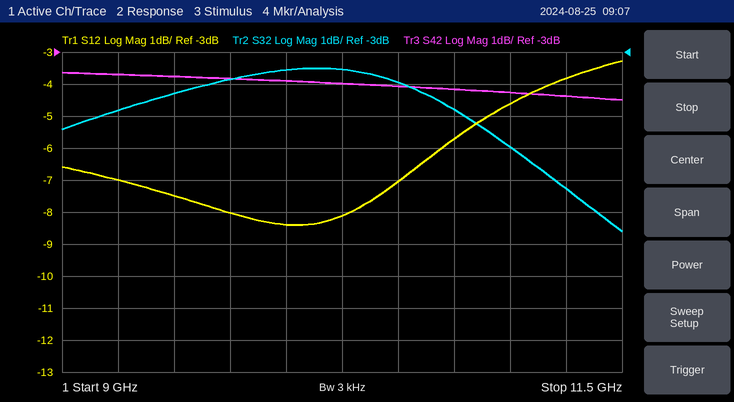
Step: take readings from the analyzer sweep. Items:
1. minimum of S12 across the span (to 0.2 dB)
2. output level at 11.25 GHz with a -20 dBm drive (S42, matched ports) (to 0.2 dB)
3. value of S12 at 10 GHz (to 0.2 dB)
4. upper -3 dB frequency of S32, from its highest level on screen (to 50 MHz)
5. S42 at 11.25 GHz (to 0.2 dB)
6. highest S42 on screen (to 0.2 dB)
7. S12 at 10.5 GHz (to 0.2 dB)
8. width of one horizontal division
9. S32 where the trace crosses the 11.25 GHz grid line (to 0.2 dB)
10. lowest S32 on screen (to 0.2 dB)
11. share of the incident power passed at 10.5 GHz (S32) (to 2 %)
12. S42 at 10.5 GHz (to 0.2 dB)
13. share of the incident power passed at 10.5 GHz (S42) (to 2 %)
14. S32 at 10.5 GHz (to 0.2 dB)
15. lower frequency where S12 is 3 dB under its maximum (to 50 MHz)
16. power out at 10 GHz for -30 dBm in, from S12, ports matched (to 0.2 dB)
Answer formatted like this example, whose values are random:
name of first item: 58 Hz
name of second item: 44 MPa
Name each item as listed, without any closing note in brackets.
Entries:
minimum of S12 across the span: -8.4 dB
output level at 11.25 GHz with a -20 dBm drive (S42, matched ports): -24.4 dBm
value of S12 at 10 GHz: -8.4 dB
upper -3 dB frequency of S32, from its highest level on screen: 11.10 GHz
S42 at 11.25 GHz: -4.4 dB
highest S42 on screen: -3.6 dB
S12 at 10.5 GHz: -7.0 dB
width of one horizontal division: 250 MHz
S32 where the trace crosses the 11.25 GHz grid line: -7.2 dB
lowest S32 on screen: -8.6 dB
share of the incident power passed at 10.5 GHz (S32): 40 %
S42 at 10.5 GHz: -4.0 dB
share of the incident power passed at 10.5 GHz (S42): 40 %
S32 at 10.5 GHz: -4.0 dB
lower frequency where S12 is 3 dB under its maximum: 10.65 GHz
power out at 10 GHz for -30 dBm in, from S12, ports matched: -38.4 dBm
